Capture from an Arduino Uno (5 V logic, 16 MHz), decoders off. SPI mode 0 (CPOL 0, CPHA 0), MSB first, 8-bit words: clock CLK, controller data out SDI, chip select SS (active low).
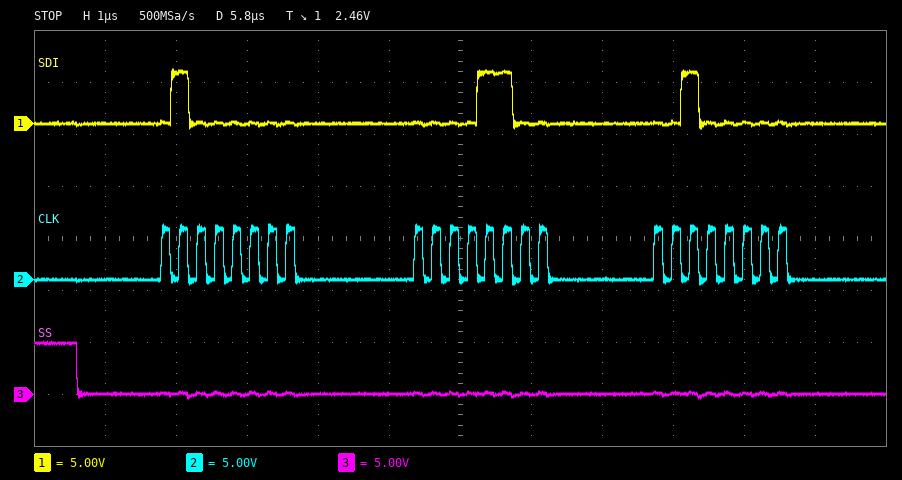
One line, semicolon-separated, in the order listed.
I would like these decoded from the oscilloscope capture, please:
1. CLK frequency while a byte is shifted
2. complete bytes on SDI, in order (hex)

4 MHz; 40 0C 20
